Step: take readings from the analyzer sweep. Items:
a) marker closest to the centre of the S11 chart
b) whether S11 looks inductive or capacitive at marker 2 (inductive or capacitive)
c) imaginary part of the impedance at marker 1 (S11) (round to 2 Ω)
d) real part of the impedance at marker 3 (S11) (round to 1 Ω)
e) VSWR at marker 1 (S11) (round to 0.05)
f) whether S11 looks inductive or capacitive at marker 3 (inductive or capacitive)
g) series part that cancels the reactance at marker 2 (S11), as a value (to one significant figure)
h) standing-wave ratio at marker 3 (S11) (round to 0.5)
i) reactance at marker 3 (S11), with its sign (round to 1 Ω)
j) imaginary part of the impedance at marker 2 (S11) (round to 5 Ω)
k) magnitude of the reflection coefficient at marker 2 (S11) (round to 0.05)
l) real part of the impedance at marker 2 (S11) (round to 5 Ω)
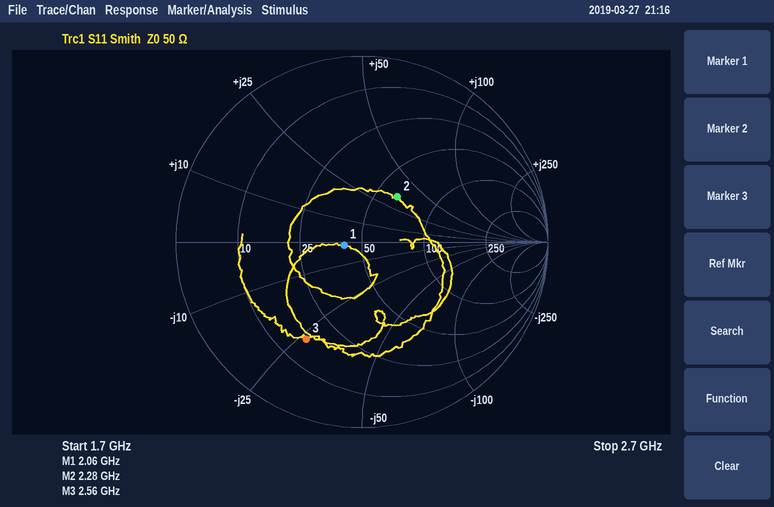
marker 1
inductive
-2 Ω
16 Ω
1.20
capacitive
2 pF
4.0
-27 Ω
+35 Ω
0.30
65 Ω
